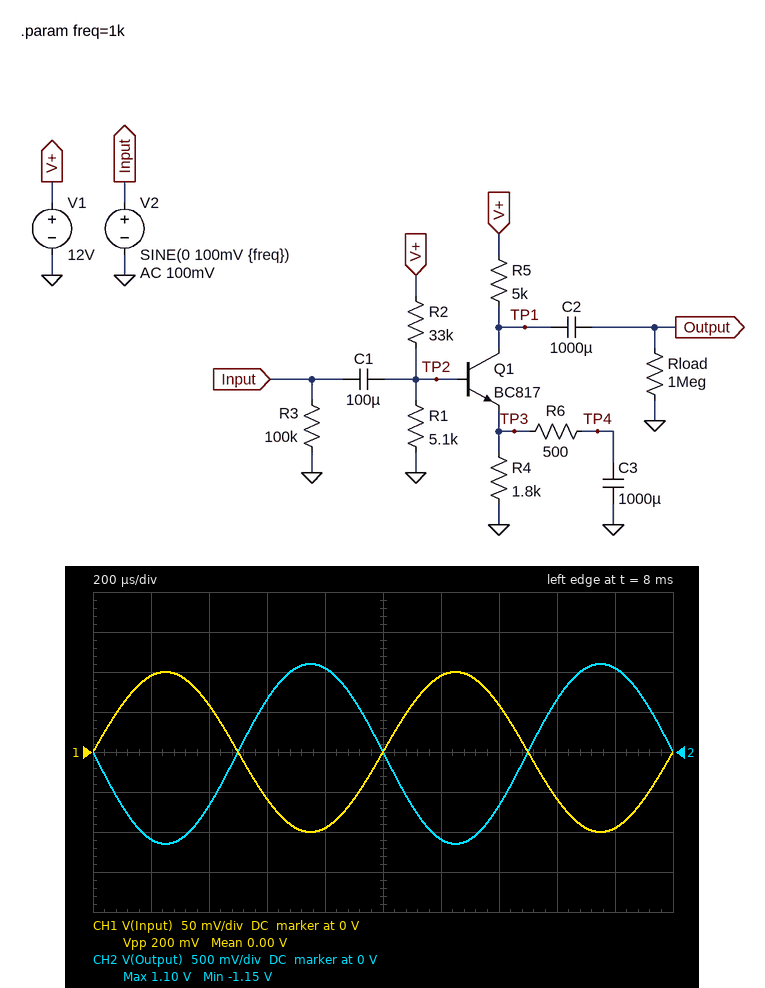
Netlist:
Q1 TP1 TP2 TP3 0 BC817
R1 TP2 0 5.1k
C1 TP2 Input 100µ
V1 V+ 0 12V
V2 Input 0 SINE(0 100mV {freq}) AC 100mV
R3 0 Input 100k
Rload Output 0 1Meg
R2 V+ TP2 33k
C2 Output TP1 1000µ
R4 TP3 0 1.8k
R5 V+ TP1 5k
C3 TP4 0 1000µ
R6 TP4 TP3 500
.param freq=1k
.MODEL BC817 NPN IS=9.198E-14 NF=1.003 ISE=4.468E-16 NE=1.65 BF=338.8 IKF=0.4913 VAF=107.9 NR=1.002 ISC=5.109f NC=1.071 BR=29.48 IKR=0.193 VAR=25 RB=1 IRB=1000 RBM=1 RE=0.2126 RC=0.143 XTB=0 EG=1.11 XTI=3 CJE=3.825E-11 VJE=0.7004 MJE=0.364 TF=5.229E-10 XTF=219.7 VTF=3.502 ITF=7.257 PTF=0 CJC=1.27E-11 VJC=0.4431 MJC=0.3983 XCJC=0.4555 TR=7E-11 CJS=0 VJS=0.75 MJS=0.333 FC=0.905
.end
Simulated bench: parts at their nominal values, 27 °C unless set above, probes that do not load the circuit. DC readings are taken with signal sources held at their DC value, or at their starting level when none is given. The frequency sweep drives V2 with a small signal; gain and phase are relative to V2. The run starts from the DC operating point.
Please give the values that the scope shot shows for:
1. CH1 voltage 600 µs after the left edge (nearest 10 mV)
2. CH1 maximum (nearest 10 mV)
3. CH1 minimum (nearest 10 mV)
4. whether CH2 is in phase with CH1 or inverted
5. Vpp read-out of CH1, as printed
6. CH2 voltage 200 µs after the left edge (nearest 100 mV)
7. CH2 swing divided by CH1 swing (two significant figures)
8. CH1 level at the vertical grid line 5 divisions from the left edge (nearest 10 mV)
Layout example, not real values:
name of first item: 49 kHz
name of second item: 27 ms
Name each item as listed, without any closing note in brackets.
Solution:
CH1 voltage 600 µs after the left edge: -60 mV
CH1 maximum: 100 mV
CH1 minimum: -100 mV
whether CH2 is in phase with CH1 or inverted: inverted
Vpp read-out of CH1, as printed: 200 mV
CH2 voltage 200 µs after the left edge: -1.1 V
CH2 swing divided by CH1 swing: 11
CH1 level at the vertical grid line 5 divisions from the left edge: 0 V
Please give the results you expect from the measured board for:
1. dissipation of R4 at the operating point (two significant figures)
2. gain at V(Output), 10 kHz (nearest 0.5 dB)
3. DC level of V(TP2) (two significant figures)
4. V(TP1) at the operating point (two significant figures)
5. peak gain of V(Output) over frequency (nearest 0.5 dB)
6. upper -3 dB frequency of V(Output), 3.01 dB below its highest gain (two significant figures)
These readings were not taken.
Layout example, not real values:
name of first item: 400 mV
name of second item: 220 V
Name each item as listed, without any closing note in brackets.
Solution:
dissipation of R4 at the operating point: 570 µW
gain at V(Output), 10 kHz: 21.0 dB
DC level of V(TP2): 1.6 V
V(TP1) at the operating point: 9.2 V
peak gain of V(Output) over frequency: 21.0 dB
upper -3 dB frequency of V(Output), 3.01 dB below its highest gain: 8.0 MHz
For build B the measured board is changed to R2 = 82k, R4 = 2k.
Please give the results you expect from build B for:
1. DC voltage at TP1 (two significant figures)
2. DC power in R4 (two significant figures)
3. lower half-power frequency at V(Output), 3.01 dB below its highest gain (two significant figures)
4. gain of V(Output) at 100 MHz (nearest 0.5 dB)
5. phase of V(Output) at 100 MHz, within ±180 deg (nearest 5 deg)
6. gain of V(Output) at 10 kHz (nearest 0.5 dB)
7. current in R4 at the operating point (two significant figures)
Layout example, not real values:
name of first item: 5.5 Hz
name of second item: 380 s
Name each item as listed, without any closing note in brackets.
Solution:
DC voltage at TP1: 12 V
DC power in R4: 14 µW
lower half-power frequency at V(Output), 3.01 dB below its highest gain: 420 mHz
gain of V(Output) at 100 MHz: 0.5 dB
phase of V(Output) at 100 MHz, within ±180 deg: 5 deg
gain of V(Output) at 10 kHz: 17.0 dB
current in R4 at the operating point: 84 µA
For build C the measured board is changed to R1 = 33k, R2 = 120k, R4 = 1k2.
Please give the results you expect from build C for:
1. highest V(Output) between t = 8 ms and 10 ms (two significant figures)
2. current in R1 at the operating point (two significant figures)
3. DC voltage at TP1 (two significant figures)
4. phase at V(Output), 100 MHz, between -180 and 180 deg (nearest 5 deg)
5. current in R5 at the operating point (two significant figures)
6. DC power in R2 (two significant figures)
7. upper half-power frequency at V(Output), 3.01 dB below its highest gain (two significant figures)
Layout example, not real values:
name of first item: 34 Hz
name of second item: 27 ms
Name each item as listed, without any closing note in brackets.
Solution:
highest V(Output) between t = 8 ms and 10 ms: 1.3 V
current in R1 at the operating point: 75 µA
DC voltage at TP1: 4.3 V
phase at V(Output), 100 MHz, between -180 and 180 deg: 15 deg
current in R5 at the operating point: 1.5 mA
DC power in R2: 760 µW
upper half-power frequency at V(Output), 3.01 dB below its highest gain: 4.9 MHz
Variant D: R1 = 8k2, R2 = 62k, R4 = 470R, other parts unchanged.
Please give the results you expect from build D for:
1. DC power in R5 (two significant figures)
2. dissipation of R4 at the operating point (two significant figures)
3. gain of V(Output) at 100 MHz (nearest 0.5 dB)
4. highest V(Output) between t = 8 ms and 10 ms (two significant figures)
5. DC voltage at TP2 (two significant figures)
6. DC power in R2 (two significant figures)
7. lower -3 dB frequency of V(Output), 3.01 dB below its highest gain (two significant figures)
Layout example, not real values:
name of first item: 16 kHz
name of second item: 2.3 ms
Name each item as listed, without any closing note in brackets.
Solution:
DC power in R5: 13 mW
dissipation of R4 at the operating point: 1.2 mW
gain of V(Output) at 100 MHz: 4.0 dB
highest V(Output) between t = 8 ms and 10 ms: 1.9 V
DC voltage at TP2: 1.4 V
DC power in R2: 1.8 mW
lower -3 dB frequency of V(Output), 3.01 dB below its highest gain: 370 mHz
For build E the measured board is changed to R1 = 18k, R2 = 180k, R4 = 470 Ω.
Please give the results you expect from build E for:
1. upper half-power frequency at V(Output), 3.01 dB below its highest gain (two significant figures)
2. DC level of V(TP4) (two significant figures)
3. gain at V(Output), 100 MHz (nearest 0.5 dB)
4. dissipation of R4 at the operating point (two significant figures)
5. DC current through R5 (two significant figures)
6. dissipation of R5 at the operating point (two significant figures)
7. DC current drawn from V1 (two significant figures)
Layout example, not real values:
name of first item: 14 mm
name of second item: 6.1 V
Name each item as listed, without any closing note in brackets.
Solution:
upper half-power frequency at V(Output), 3.01 dB below its highest gain: 7.4 MHz
DC level of V(TP4): 450 mV
gain at V(Output), 100 MHz: 4.5 dB
dissipation of R4 at the operating point: 430 µW
DC current through R5: 950 µA
dissipation of R5 at the operating point: 4.5 mW
DC current drawn from V1: 1.0 mA
